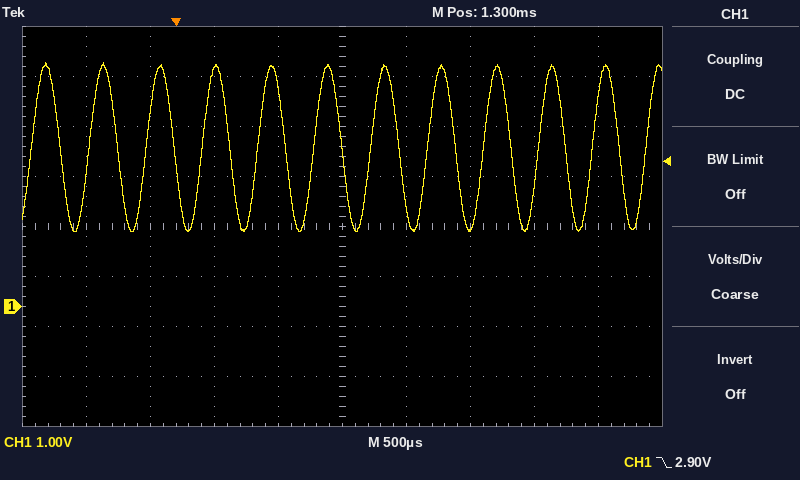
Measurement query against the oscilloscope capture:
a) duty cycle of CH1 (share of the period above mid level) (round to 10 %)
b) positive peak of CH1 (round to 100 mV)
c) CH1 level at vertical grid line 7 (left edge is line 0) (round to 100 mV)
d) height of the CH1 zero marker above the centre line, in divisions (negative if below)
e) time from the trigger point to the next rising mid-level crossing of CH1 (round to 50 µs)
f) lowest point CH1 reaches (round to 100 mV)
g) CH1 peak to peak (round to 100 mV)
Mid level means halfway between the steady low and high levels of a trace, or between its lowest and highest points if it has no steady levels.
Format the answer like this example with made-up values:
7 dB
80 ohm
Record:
50 %
4.9 V
1.6 V
-1.6 div
200 µs
1.5 V
3.4 V
